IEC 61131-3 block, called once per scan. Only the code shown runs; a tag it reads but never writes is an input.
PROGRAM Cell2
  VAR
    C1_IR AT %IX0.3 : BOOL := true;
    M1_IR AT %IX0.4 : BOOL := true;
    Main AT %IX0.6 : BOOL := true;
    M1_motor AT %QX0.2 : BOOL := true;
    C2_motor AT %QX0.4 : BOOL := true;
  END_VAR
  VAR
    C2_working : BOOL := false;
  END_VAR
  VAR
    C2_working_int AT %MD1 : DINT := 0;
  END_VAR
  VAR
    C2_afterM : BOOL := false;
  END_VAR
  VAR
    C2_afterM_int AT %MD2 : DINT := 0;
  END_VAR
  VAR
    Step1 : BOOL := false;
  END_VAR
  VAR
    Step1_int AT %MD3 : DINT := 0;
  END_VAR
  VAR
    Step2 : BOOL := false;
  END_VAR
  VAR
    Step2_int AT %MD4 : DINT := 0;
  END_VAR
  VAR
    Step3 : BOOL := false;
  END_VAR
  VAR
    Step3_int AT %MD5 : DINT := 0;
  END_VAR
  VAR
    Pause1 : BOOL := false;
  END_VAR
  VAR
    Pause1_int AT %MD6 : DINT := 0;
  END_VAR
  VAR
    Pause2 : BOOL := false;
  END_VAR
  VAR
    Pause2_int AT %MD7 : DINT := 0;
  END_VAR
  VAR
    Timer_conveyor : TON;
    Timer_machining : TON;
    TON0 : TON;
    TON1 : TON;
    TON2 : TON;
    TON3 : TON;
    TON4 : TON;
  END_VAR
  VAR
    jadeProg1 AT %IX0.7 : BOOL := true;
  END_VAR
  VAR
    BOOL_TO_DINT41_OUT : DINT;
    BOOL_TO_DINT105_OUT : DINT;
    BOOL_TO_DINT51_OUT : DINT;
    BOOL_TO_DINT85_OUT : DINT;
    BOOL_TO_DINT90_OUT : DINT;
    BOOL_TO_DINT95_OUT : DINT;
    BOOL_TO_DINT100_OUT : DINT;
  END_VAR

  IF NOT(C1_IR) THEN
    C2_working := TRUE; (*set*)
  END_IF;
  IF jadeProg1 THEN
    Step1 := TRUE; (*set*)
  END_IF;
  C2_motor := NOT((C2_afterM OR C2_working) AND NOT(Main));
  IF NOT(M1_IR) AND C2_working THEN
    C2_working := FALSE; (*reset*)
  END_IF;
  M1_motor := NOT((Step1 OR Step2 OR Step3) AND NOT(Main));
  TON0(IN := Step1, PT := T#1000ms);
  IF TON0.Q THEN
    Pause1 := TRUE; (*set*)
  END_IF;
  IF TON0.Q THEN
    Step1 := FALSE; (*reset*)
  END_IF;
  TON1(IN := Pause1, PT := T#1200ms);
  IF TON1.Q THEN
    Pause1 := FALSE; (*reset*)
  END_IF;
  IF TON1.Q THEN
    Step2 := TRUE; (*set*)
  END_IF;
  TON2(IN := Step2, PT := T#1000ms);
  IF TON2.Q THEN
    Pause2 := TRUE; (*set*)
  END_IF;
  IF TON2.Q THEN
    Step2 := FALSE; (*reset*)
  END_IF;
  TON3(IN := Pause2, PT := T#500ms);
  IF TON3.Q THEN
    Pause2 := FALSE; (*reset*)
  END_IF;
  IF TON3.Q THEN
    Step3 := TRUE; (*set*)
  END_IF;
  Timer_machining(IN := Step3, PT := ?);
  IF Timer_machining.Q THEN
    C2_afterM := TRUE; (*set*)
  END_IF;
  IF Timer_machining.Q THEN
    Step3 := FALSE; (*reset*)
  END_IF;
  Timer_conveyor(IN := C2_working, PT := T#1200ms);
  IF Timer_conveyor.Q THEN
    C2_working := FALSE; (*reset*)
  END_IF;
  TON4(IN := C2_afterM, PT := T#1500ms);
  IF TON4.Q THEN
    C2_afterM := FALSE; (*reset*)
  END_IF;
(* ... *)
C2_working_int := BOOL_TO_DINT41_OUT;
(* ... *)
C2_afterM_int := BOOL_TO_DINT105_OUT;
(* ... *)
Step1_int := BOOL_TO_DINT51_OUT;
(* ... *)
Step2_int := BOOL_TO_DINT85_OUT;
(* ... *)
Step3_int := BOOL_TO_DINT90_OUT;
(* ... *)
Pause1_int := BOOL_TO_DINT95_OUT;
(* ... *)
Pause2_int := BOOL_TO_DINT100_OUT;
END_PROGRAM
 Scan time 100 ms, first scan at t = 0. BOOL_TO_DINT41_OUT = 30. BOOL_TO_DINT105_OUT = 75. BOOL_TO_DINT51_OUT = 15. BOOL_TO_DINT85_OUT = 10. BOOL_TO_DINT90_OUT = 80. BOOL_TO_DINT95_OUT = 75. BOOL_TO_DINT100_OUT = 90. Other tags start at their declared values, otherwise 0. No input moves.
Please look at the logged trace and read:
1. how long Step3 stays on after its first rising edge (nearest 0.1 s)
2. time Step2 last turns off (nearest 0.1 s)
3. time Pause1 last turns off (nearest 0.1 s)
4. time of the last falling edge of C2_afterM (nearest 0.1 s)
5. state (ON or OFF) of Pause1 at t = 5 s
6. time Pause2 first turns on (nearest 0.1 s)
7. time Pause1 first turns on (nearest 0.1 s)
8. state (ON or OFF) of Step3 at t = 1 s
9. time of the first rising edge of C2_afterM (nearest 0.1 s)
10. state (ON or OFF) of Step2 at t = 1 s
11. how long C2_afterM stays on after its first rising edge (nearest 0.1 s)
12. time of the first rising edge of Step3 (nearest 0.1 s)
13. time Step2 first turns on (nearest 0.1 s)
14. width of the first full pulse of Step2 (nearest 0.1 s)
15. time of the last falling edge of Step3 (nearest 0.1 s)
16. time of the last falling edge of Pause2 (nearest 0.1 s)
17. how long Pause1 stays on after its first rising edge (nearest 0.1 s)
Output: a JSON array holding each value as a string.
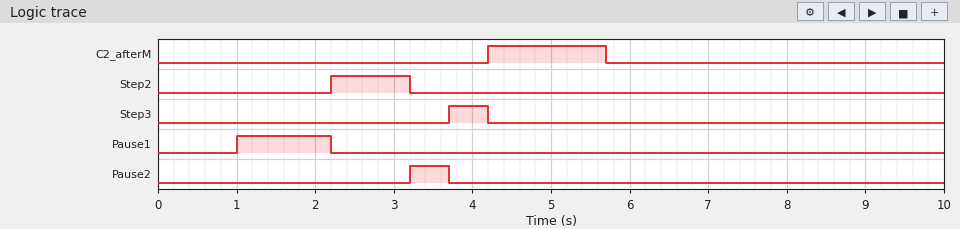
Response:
["0.5 s", "3.2 s", "2.2 s", "5.7 s", "OFF", "3.2 s", "1.0 s", "OFF", "4.2 s", "OFF", "1.5 s", "3.7 s", "2.2 s", "1.0 s", "4.2 s", "3.7 s", "1.2 s"]
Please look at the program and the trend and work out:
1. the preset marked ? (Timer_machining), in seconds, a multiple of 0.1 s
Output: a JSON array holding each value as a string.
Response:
["0.5 s"]
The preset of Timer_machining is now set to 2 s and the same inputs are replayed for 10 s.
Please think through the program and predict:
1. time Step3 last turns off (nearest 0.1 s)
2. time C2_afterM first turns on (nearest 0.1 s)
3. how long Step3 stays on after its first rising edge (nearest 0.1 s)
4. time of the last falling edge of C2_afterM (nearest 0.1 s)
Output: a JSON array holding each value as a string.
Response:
["5.7 s", "5.7 s", "2.0 s", "7.2 s"]
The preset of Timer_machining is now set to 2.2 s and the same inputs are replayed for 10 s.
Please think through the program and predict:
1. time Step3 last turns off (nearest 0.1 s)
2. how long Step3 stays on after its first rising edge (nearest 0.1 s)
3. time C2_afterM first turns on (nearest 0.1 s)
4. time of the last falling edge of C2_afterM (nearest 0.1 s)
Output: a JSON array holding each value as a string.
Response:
["5.9 s", "2.2 s", "5.9 s", "7.4 s"]
